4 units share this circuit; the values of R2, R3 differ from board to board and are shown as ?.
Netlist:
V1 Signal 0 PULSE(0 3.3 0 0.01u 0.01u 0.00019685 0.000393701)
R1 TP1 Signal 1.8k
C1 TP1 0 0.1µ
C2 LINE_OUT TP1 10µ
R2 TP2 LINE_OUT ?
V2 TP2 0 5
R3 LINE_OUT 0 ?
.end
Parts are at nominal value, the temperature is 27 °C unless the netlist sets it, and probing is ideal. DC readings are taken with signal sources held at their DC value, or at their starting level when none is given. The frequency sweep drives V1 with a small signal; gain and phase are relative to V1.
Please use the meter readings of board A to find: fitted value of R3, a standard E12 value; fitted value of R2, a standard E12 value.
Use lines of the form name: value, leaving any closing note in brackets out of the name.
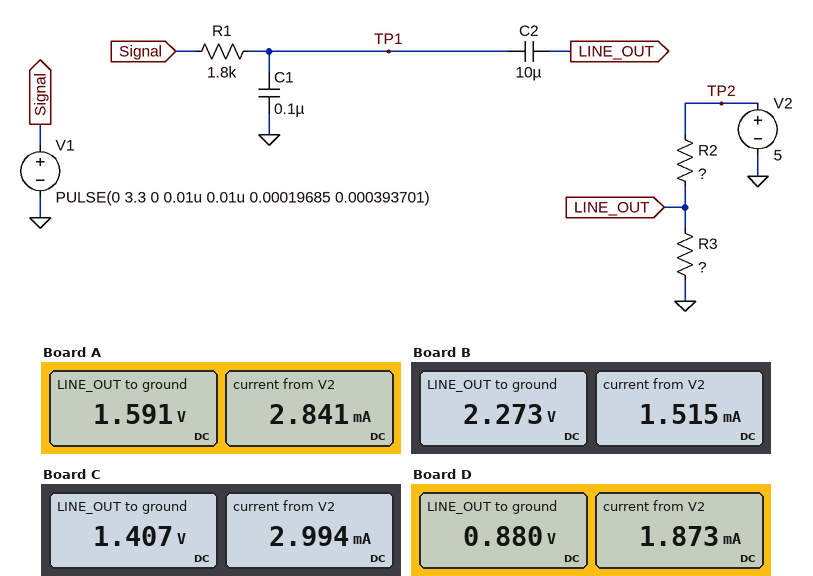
fitted value of R3, a standard E12 value: 560 Ω
fitted value of R2, a standard E12 value: 1.2 kΩ
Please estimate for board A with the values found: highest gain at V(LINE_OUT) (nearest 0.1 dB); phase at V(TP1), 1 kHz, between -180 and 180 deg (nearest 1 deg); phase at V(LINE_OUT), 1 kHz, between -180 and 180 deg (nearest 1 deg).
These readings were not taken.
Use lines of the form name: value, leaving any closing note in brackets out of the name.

highest gain at V(LINE_OUT): -15.2 dB
phase at V(TP1), 1 kHz, between -180 and 180 deg: -13 deg
phase at V(LINE_OUT), 1 kHz, between -180 and 180 deg: -11 deg
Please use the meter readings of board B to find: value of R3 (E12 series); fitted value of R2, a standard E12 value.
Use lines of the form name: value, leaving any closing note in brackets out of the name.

value of R3: 1.5 kΩ
fitted value of R2, a standard E12 value: 1.8 kΩ
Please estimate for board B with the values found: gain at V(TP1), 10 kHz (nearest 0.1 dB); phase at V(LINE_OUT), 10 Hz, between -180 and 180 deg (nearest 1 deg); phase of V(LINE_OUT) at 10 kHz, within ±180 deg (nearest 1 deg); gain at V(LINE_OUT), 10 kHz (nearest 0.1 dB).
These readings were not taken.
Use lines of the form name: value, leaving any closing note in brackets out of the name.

gain at V(TP1), 10 kHz: -21.4 dB
phase at V(LINE_OUT), 10 Hz, between -180 and 180 deg: 31 deg
phase of V(LINE_OUT) at 10 kHz, within ±180 deg: -74 deg
gain at V(LINE_OUT), 10 kHz: -21.4 dB
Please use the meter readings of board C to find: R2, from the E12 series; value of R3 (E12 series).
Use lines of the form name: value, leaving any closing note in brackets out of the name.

R2, from the E12 series: 1.2 kΩ
value of R3: 470 Ω
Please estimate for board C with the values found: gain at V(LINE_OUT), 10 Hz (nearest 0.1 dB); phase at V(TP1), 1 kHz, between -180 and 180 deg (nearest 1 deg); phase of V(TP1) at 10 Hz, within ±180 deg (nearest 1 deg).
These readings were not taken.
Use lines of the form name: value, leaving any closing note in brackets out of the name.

gain at V(LINE_OUT), 10 Hz: -18.0 dB
phase at V(TP1), 1 kHz, between -180 and 180 deg: -12 deg
phase of V(TP1) at 10 Hz, within ±180 deg: -42 deg
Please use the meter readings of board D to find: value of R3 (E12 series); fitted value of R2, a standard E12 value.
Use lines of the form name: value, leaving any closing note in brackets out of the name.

value of R3: 470 Ω
fitted value of R2, a standard E12 value: 2.2 kΩ
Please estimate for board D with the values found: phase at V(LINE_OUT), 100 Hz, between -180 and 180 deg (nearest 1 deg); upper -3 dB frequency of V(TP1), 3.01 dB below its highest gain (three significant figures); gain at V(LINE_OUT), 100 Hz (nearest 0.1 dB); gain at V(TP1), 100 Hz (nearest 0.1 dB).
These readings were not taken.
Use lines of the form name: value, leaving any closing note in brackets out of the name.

phase at V(LINE_OUT), 100 Hz, between -180 and 180 deg: 3 deg
upper -3 dB frequency of V(TP1), 3.01 dB below its highest gain: 7.46 Hz
gain at V(LINE_OUT), 100 Hz: -15.1 dB
gain at V(TP1), 100 Hz: -14.4 dB
